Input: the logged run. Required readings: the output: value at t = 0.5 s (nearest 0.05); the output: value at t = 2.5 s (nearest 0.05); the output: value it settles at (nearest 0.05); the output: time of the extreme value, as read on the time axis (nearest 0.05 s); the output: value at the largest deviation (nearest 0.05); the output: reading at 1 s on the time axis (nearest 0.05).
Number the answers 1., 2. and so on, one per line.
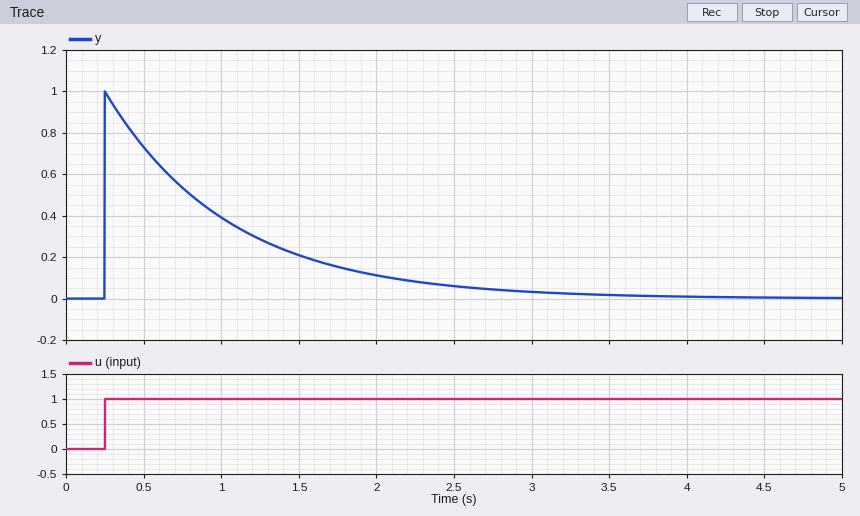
1. 0.75
2. 0.05
3. 0.00
4. 0.25 s
5. 1.00
6. 0.40
